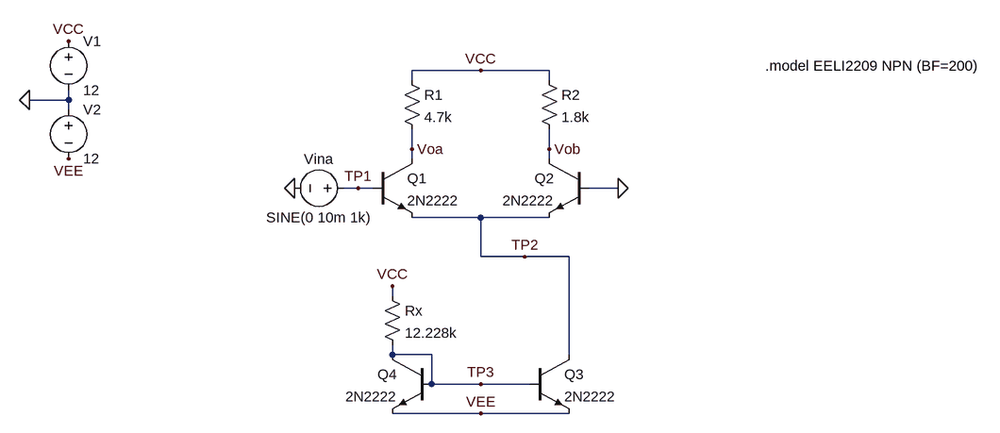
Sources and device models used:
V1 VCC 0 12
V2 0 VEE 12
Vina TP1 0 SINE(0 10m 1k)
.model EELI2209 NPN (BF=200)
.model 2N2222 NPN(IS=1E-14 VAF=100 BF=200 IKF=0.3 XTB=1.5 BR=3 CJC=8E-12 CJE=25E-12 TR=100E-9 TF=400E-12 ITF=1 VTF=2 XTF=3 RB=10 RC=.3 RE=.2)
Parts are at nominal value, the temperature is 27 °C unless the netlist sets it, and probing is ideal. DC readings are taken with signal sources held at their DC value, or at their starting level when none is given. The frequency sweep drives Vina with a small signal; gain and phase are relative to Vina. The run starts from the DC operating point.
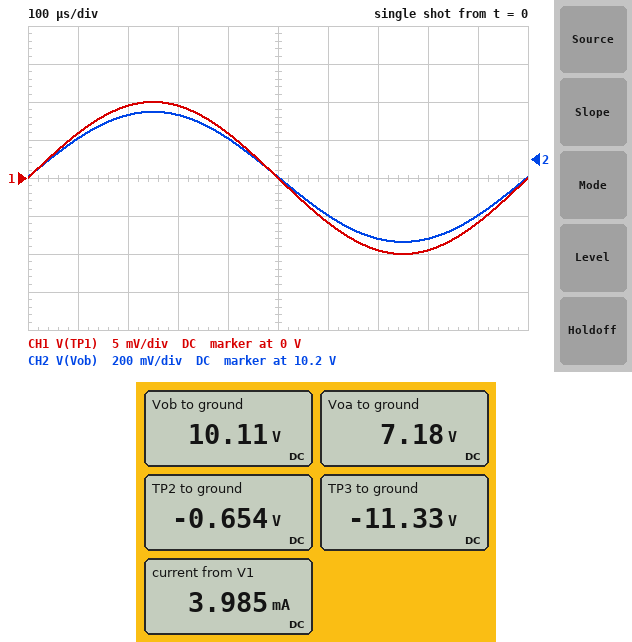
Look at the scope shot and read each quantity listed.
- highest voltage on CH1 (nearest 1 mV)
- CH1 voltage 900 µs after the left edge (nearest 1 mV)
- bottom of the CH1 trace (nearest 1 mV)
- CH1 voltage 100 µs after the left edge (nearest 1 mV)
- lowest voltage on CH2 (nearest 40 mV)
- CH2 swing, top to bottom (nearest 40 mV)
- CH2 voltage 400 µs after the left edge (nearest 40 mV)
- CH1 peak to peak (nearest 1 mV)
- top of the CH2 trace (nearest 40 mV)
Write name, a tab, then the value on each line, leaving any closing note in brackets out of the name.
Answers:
highest voltage on CH1	10 mV
CH1 voltage 900 µs after the left edge	-6 mV
bottom of the CH1 trace	-10 mV
CH1 voltage 100 µs after the left edge	6 mV
lowest voltage on CH2	9.76 V
CH2 swing, top to bottom	680 mV
CH2 voltage 400 µs after the left edge	10.32 V
CH1 peak to peak	20 mV
top of the CH2 trace	10.44 V
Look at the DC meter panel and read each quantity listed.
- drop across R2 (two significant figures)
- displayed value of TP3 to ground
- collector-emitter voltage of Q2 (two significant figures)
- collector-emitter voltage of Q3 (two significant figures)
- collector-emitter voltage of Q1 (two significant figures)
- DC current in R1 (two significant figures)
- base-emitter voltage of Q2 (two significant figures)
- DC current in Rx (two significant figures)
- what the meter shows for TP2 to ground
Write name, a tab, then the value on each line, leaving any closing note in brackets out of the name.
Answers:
drop across R2	1.9 V
displayed value of TP3 to ground	-11.33 V
collector-emitter voltage of Q2	11 V
collector-emitter voltage of Q3	11 V
collector-emitter voltage of Q1	7.8 V
DC current in R1	1.0 mA
base-emitter voltage of Q2	650 mV
DC current in Rx	1.9 mA
what the meter shows for TP2 to ground	-0.654 V
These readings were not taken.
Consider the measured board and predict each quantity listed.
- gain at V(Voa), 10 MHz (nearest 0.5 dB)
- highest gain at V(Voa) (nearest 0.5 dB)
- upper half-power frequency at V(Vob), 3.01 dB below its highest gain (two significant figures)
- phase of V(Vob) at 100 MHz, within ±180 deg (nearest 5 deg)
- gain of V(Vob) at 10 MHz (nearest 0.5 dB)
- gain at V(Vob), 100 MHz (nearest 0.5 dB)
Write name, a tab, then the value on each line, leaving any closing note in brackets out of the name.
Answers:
gain at V(Voa), 10 MHz	34.5 dB
highest gain at V(Voa)	39.0 dB
upper half-power frequency at V(Vob), 3.01 dB below its highest gain	16 MHz
phase of V(Vob) at 100 MHz, within ±180 deg	-90 deg
gain of V(Vob) at 10 MHz	29.0 dB
gain at V(Vob), 100 MHz	15.5 dB
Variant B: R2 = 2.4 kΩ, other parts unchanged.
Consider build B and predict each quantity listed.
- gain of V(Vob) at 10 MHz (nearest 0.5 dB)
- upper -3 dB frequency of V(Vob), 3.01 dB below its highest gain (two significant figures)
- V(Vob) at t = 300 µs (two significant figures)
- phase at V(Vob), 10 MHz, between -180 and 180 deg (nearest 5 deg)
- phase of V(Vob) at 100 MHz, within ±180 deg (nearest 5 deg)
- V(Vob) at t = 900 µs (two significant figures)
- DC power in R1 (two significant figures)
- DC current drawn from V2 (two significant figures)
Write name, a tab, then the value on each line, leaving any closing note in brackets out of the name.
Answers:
gain of V(Vob) at 10 MHz	31.0 dB
upper -3 dB frequency of V(Vob), 3.01 dB below its highest gain	13 MHz
V(Vob) at t = 300 µs	9.9 V
phase at V(Vob), 10 MHz, between -180 and 180 deg	-35 deg
phase of V(Vob) at 100 MHz, within ±180 deg	-95 deg
V(Vob) at t = 900 µs	9.2 V
DC power in R1	5.0 mW
DC current drawn from V2	4.0 mA
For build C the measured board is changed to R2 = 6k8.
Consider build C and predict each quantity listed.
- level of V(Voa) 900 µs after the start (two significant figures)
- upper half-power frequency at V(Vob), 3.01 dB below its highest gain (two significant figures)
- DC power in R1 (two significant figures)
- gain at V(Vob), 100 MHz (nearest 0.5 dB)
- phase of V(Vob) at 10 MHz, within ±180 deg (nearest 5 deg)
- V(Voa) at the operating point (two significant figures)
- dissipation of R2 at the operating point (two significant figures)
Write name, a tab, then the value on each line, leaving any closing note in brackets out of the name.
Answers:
level of V(Voa) 900 µs after the start	7.6 V
upper half-power frequency at V(Vob), 3.01 dB below its highest gain	4.6 MHz
DC power in R1	5.2 mW
gain at V(Vob), 100 MHz	14.0 dB
phase of V(Vob) at 10 MHz, within ±180 deg	-70 deg
V(Voa) at the operating point	7.1 V
dissipation of R2 at the operating point	7.2 mW
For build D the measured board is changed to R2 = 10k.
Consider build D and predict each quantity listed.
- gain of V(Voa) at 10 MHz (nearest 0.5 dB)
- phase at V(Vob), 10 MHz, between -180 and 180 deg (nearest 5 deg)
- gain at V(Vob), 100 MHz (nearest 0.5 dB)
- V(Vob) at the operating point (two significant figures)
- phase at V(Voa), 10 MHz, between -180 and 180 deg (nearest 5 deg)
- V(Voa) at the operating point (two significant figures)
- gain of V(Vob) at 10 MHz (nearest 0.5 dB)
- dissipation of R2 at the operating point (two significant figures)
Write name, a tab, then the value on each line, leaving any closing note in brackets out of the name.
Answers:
gain of V(Voa) at 10 MHz	33.5 dB
phase at V(Vob), 10 MHz, between -180 and 180 deg	-80 deg
gain at V(Vob), 100 MHz	11.5 dB
V(Vob) at the operating point	1.9 V
phase at V(Voa), 10 MHz, between -180 and 180 deg	125 deg
V(Voa) at the operating point	7.0 V
gain of V(Vob) at 10 MHz	32.5 dB
dissipation of R2 at the operating point	10 mW
